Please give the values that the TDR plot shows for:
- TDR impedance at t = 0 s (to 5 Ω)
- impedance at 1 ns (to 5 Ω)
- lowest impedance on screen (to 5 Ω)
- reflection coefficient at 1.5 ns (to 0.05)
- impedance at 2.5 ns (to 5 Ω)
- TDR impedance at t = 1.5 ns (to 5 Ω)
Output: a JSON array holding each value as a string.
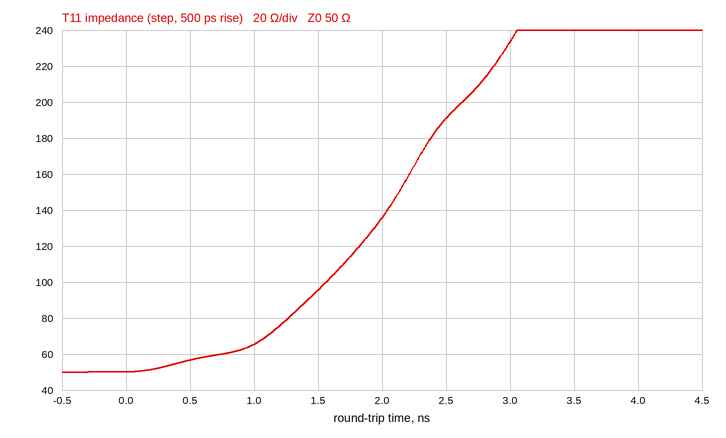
["50 Ω", "65 Ω", "50 Ω", "+0.30", "190 Ω", "95 Ω"]
